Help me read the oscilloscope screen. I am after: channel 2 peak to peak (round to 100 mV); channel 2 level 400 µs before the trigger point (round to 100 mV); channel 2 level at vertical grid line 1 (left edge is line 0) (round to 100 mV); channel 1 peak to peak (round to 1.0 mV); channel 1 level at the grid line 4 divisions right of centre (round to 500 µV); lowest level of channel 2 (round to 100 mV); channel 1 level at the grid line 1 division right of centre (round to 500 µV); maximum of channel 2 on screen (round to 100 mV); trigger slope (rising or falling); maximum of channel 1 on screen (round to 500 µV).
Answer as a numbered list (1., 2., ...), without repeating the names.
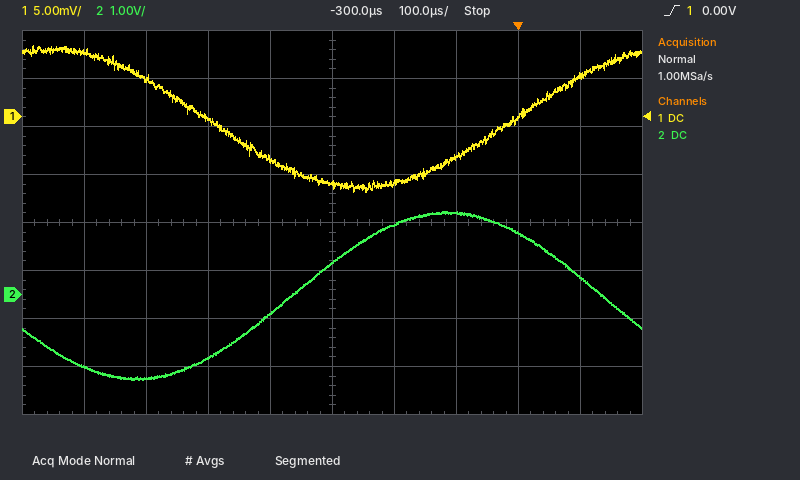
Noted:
1. 3.5 V
2. -400 mV
3. -1.5 V
4. 15.0 mV
5. 4.5 mV
6. -1.8 V
7. -7.0 mV
8. 1.7 V
9. rising
10. 7.5 mV
